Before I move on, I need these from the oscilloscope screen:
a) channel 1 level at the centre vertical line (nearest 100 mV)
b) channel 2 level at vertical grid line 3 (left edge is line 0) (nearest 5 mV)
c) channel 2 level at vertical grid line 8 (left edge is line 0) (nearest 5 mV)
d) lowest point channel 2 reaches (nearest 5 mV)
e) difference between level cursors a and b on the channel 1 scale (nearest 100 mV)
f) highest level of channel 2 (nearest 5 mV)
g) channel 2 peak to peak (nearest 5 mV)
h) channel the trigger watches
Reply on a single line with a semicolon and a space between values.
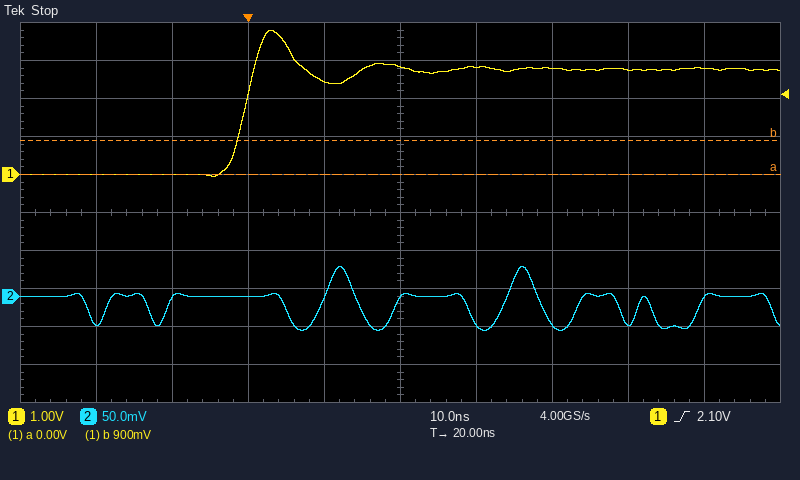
2.8 V; 0 mV; -35 mV; -45 mV; 900 mV; 40 mV; 85 mV; channel 1
